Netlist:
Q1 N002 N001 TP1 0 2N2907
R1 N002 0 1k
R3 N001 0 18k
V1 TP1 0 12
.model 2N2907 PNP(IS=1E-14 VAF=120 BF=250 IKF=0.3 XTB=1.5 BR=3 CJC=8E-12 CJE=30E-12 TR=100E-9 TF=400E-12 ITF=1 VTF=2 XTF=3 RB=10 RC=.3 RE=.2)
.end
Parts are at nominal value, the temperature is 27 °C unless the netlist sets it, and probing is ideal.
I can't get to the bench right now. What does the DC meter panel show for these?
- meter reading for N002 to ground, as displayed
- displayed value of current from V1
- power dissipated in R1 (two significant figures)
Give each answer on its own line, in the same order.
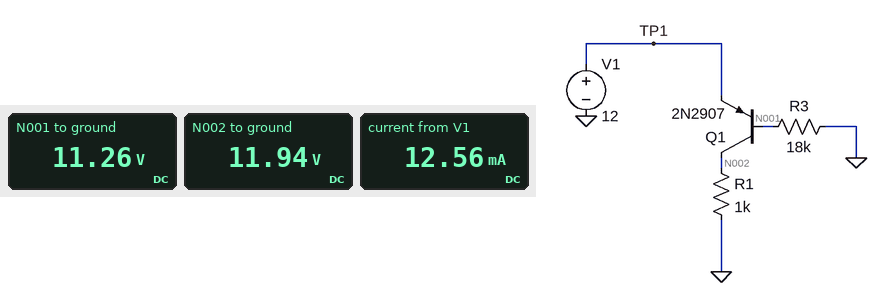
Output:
11.94 V
12.56 mA
140 mW
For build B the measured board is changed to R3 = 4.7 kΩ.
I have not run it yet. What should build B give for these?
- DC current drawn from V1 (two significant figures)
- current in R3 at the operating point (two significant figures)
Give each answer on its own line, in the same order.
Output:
14 mA
2.4 mA
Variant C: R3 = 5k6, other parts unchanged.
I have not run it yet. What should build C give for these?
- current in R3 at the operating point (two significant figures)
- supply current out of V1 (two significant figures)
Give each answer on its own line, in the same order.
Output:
2.0 mA
14 mA
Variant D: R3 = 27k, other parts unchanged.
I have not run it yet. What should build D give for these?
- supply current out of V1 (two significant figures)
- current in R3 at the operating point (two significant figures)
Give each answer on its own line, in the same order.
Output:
12 mA
420 µA
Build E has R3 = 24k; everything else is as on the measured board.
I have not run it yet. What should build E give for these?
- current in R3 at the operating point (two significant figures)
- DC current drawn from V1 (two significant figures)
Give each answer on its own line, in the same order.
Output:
470 µA
12 mA
